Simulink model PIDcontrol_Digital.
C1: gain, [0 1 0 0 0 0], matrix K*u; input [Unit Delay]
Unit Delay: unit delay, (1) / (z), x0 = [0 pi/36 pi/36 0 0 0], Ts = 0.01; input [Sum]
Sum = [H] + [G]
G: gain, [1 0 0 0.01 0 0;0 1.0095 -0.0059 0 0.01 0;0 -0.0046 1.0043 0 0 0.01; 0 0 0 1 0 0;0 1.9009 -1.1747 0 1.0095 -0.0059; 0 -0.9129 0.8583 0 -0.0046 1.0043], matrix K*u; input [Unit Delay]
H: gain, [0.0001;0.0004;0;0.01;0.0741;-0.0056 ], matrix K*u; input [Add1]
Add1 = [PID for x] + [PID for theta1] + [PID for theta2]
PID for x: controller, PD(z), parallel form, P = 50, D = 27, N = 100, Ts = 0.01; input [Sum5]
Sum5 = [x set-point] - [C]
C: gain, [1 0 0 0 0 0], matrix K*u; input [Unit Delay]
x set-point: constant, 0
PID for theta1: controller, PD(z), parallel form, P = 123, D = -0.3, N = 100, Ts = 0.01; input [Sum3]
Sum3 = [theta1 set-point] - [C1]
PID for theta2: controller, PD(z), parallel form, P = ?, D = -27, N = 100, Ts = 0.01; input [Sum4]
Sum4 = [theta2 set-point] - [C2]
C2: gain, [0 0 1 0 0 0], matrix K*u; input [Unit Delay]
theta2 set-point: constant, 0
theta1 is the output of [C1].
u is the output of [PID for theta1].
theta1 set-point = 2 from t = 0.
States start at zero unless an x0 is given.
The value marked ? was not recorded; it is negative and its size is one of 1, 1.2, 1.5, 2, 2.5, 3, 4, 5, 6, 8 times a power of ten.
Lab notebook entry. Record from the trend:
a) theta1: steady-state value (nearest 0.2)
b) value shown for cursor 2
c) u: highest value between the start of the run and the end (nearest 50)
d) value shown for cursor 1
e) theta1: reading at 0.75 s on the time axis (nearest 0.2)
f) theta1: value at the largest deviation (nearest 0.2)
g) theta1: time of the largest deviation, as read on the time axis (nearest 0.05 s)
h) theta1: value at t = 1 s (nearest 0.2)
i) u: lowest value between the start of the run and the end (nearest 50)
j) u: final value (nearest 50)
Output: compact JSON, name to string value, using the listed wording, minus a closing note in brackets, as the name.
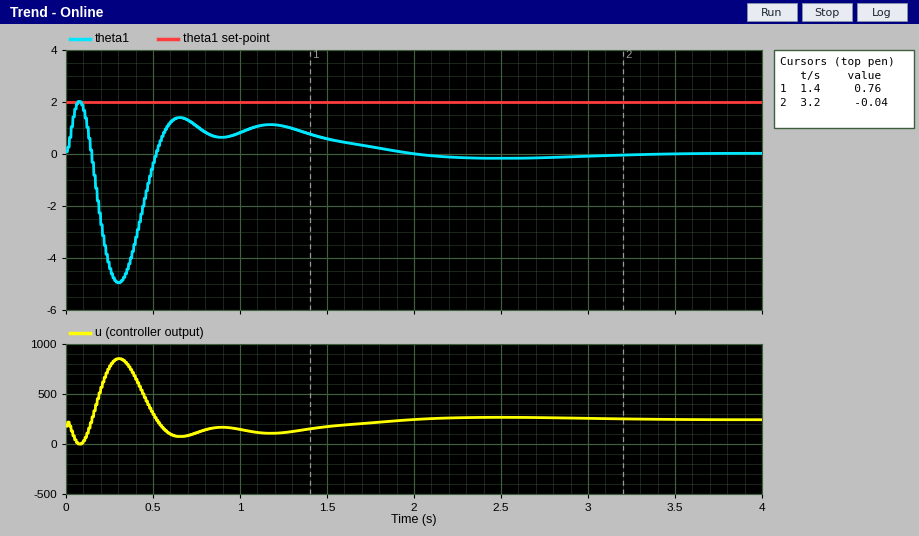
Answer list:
{"theta1: steady-state value": "0.0", "value shown for cursor 2": "-0.04", "u: highest value between the start of the run and the end": "850", "value shown for cursor 1": "0.76", "theta1: reading at 0.75 s on the time axis": "1.0", "theta1: value at the largest deviation": "-5.0", "theta1: time of the largest deviation, as read on the time axis": "0.30 s", "theta1: value at t = 1 s": "0.8", "u: lowest value between the start of the run and the end": "0", "u: final value": "250"}
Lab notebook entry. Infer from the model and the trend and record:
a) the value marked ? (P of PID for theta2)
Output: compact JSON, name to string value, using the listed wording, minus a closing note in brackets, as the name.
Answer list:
{"the value marked ?": "-250"}
